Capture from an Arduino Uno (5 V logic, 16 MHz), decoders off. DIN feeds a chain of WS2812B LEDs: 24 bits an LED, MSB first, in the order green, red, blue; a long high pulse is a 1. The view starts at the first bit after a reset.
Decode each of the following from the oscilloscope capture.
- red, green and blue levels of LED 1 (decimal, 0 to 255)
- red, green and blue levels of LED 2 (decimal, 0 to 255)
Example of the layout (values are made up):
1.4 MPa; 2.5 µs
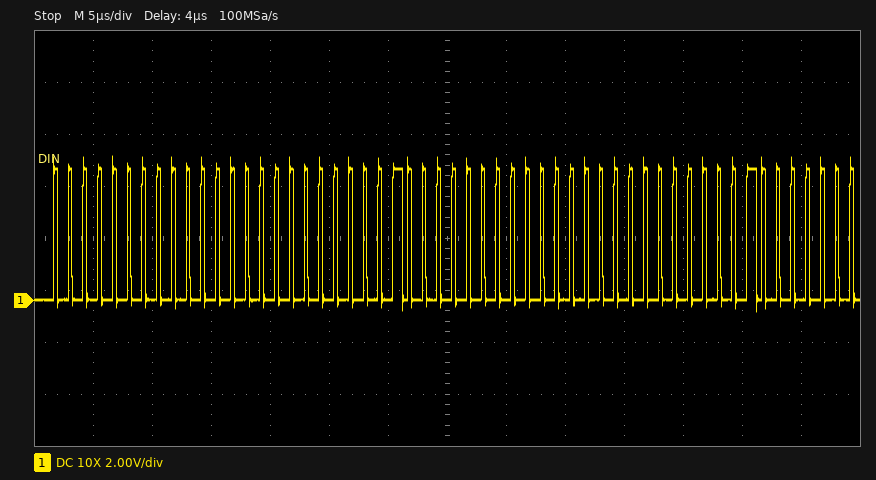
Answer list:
0, 0, 1; 0, 0, 1
